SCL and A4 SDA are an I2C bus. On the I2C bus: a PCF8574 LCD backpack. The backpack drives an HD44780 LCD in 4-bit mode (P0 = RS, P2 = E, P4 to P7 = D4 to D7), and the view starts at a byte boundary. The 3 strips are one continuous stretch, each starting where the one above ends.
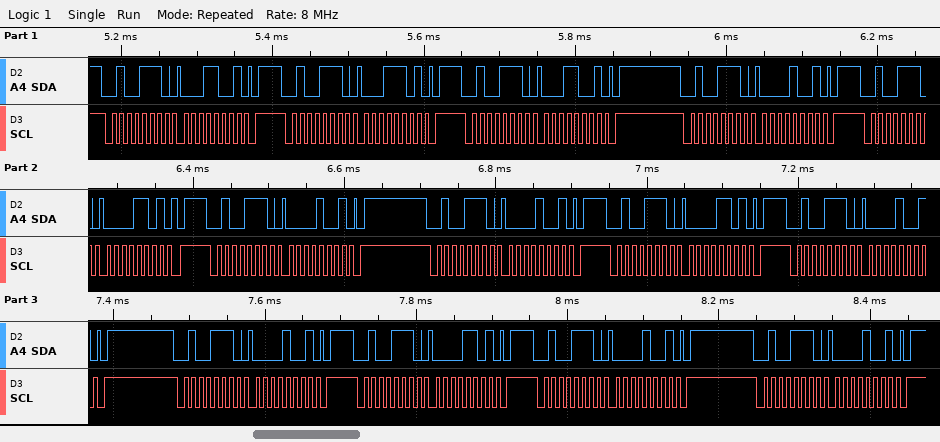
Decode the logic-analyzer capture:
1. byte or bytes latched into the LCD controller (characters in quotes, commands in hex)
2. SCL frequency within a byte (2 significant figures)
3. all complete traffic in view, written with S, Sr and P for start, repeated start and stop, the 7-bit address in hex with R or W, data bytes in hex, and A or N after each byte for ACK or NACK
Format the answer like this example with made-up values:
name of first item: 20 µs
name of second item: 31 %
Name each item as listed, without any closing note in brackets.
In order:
byte or bytes latched into the LCD controller: data 0x10 data 0x00
SCL frequency within a byte: 100 kHz
all complete traffic in view, written with S, Sr and P for start, repeated start and stop, the 7-bit address in hex with R or W, data bytes in hex, and A or N after each byte for ACK or NACK: S 27W A 19 A P S 27W A 1D A P S 27W A 19 A P S 27W A 09 A P S 27W A 0D A P S 27W A 09 A P S 27W A 09 A P S 27W A 0D A P S 27W A 09 A P S 27W A 09 A P S 27W A 0D A P S 27W A 09 A P S 27W A 09 A P
